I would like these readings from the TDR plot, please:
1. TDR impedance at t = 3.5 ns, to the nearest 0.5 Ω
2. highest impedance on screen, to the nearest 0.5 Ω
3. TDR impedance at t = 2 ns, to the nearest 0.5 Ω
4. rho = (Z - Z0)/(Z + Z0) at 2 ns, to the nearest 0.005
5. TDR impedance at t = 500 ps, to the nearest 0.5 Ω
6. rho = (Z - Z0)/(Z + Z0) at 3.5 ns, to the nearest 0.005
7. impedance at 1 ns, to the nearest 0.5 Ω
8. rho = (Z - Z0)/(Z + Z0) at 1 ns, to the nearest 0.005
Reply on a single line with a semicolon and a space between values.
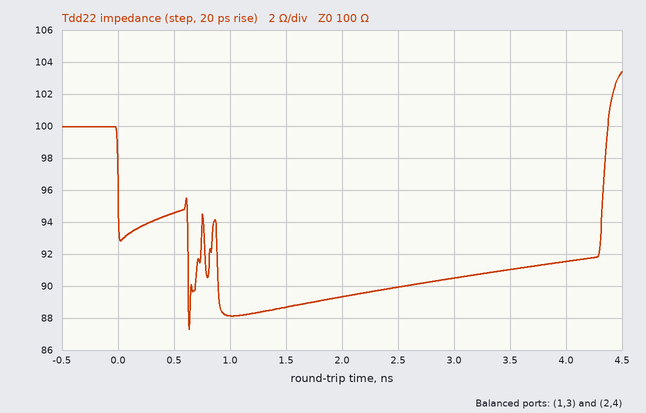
91.0 Ω; 103.5 Ω; 89.5 Ω; -0.055; 94.5 Ω; -0.045; 88.0 Ω; -0.065
